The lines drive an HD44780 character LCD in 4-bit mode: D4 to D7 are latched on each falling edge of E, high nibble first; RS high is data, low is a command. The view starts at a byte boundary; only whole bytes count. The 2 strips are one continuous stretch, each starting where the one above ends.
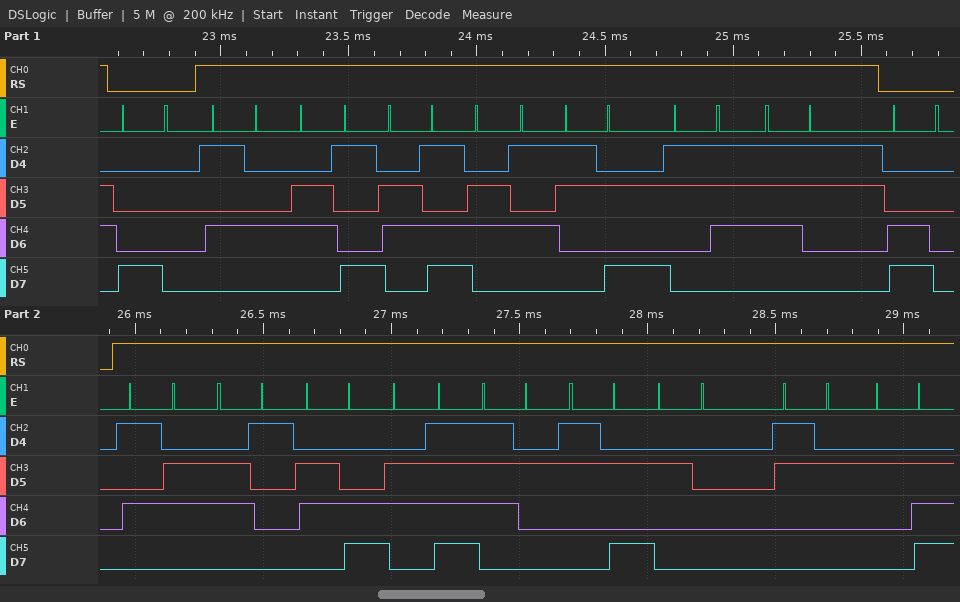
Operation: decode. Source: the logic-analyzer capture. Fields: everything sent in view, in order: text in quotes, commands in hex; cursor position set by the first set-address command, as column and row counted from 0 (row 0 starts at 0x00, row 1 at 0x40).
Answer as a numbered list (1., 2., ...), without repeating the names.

1. 0x80 "Time:7s" 0xC0 "Valor: 2."
2. column 0, row 0
